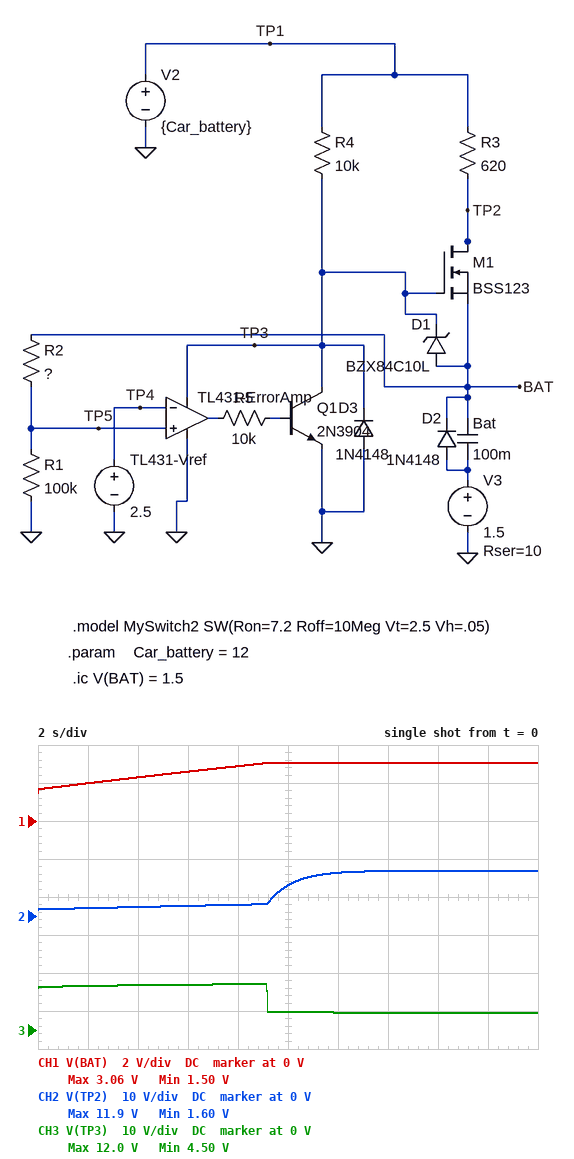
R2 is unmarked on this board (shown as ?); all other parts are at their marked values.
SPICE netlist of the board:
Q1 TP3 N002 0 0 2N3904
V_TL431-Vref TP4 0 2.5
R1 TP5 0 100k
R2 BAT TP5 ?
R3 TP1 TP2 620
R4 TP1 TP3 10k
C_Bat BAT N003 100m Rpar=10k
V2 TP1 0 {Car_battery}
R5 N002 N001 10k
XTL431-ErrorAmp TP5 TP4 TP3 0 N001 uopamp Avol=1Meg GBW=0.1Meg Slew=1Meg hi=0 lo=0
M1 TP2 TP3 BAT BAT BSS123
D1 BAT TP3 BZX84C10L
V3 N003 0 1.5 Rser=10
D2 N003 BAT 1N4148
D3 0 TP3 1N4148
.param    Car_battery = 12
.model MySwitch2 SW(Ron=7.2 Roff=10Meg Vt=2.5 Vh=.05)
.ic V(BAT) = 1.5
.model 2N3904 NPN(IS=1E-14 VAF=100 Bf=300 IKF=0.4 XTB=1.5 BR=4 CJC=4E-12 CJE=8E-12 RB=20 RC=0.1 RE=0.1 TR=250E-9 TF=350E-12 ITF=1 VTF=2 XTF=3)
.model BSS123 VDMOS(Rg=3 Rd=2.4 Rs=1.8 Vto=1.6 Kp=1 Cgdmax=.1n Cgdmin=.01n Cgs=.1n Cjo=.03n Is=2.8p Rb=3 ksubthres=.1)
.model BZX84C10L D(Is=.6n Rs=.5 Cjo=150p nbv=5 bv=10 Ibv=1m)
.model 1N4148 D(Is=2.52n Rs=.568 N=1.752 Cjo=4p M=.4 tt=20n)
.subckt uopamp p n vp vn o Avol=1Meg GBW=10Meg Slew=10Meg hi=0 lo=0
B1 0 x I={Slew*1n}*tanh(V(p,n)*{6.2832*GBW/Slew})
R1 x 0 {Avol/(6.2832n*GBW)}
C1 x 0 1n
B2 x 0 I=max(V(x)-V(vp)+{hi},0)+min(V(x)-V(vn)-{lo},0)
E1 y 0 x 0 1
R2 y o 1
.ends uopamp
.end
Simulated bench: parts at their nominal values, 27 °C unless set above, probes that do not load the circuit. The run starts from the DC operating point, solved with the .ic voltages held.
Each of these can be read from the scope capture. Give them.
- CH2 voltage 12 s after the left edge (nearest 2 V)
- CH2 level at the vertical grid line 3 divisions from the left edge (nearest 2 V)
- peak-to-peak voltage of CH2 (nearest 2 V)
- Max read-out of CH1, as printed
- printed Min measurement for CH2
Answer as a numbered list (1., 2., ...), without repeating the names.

1. 12 V
2. 2 V
3. 10 V
4. 3.06 V
5. 1.60 V
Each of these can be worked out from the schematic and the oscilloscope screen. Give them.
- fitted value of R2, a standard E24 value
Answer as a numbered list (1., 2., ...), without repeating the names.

1. 22 kΩ
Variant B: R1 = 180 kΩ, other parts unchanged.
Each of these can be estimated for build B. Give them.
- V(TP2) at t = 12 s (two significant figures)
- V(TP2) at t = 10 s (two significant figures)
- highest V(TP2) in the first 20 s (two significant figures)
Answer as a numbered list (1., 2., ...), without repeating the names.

1. 12 V
2. 11 V
3. 12 V
